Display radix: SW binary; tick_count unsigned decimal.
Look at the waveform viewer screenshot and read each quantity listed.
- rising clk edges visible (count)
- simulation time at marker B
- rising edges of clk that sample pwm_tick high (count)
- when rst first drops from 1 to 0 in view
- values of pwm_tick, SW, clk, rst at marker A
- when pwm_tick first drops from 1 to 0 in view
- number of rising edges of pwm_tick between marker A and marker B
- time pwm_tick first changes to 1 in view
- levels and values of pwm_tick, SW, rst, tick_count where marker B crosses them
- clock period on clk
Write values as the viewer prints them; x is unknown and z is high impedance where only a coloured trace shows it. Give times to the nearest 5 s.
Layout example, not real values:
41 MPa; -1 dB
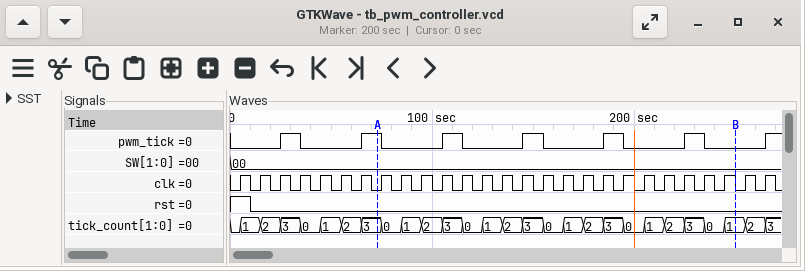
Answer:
27; 250 s; 6; 10 s; pwm_tick=1, SW=00, clk=0, rst=0; 35 s; 4; 25 s; pwm_tick=0, SW=00, rst=0, tick_count=1; 10 s
